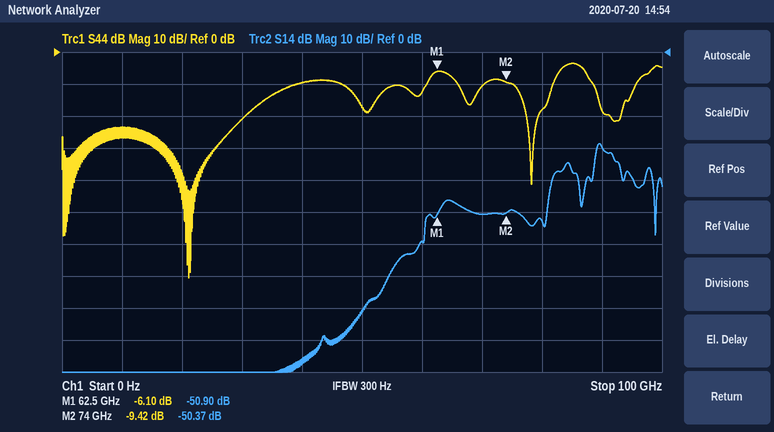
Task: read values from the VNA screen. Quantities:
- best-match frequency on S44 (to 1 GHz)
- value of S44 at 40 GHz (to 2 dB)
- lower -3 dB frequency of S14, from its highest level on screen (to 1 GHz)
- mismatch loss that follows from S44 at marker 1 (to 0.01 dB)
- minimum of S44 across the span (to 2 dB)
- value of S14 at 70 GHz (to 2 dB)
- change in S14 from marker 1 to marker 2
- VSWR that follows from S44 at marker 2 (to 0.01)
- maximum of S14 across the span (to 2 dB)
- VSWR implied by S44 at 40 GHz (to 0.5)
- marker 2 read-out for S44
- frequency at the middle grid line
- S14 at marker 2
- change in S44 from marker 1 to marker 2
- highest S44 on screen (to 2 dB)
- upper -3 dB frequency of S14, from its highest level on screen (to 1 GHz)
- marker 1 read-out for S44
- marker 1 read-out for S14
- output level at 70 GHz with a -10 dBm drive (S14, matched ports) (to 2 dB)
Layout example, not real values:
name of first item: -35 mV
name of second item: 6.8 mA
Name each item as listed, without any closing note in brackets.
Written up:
best-match frequency on S44: 21 GHz
value of S44 at 40 GHz: -10 dB
lower -3 dB frequency of S14, from its highest level on screen: 89 GHz
mismatch loss that follows from S44 at marker 1: 1.22 dB
minimum of S44 across the span: -70 dB
value of S14 at 70 GHz: -50 dB
change in S14 from marker 1 to marker 2: 0.53 dB
VSWR that follows from S44 at marker 2: 2.02
maximum of S14 across the span: -28 dB
VSWR implied by S44 at 40 GHz: 2.0
marker 2 read-out for S44: -9.42 dB
frequency at the middle grid line: 50 GHz
S14 at marker 2: -50.37 dB
change in S44 from marker 1 to marker 2: -3.32 dB
highest S44 on screen: -4 dB
upper -3 dB frequency of S14, from its highest level on screen: 91 GHz
marker 1 read-out for S44: -6.10 dB
marker 1 read-out for S14: -50.90 dB
output level at 70 GHz with a -10 dBm drive (S14, matched ports): -60 dBm
